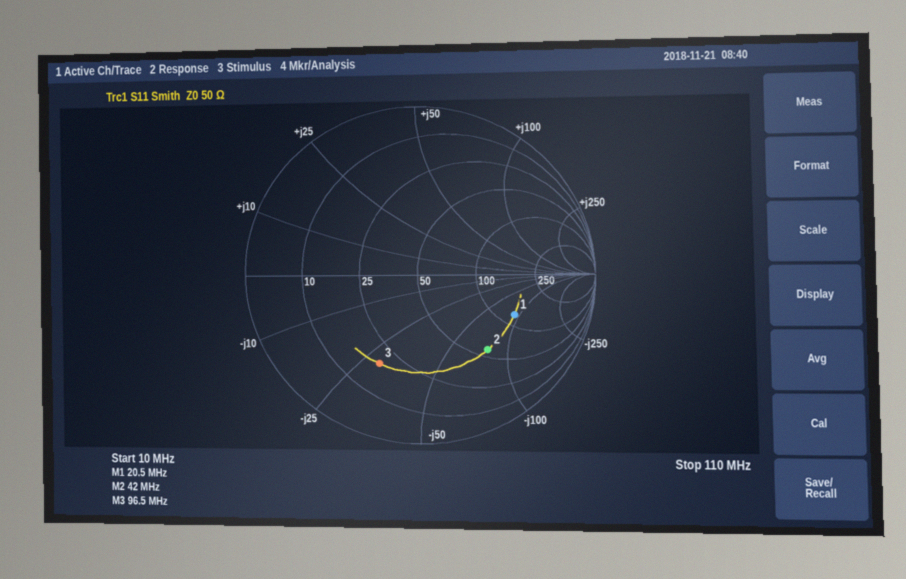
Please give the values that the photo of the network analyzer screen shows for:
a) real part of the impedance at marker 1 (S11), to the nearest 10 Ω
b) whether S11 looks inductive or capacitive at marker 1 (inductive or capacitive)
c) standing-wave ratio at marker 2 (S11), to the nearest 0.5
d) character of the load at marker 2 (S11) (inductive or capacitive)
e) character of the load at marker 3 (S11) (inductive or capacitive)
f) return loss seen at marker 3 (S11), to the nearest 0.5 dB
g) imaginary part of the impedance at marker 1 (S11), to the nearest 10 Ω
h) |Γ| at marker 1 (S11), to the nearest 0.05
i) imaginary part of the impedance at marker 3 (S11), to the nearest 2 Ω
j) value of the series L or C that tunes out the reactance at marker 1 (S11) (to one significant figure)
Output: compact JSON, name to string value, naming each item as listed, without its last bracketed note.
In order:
{"real part of the impedance at marker 1 (S11), to the nearest 10 Ω": "120 Ω", "whether S11 looks inductive or capacitive at marker 1": "capacitive", "standing-wave ratio at marker 2 (S11), to the nearest 0.5": "4.0", "character of the load at marker 2 (S11)": "capacitive", "character of the load at marker 3 (S11)": "capacitive", "return loss seen at marker 3 (S11), to the nearest 0.5 dB": "5.0 dB", "imaginary part of the impedance at marker 1 (S11), to the nearest 10 Ω": "-90 Ω", "|Γ| at marker 1 (S11), to the nearest 0.05": "0.60", "imaginary part of the impedance at marker 3 (S11), to the nearest 2 Ω": "-30 Ω", "value of the series L or C that tunes out the reactance at marker 1 (S11)": "700 nH"}
